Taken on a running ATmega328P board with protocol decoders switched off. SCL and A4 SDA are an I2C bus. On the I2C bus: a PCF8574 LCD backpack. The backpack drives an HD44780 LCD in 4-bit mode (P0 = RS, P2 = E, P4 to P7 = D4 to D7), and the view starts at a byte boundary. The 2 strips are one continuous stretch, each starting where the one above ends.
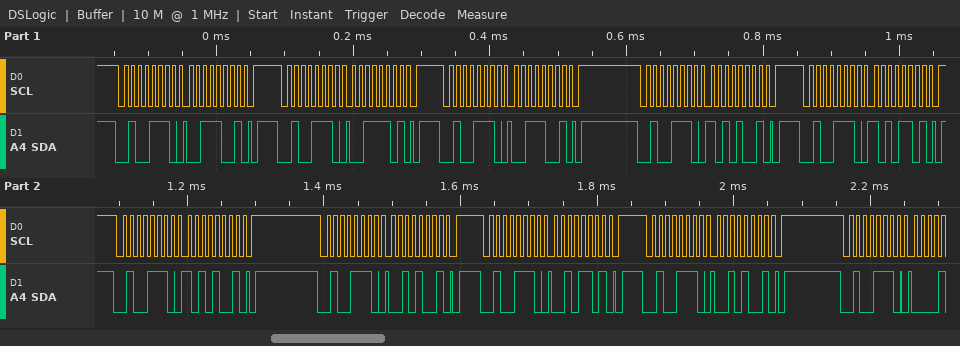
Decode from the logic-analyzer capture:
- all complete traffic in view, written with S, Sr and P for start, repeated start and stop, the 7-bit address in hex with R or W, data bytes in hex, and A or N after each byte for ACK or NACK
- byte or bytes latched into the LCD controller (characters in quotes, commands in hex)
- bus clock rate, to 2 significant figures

S 27W A 39 A P S 27W A 3D A P S 27W A 39 A P S 27W A A9 A P S 27W A AD A P S 27W A A9 A P S 27W A 29 A P S 27W A 2D A P S 27W A 29 A P S 27W A
':'
100 kHz
